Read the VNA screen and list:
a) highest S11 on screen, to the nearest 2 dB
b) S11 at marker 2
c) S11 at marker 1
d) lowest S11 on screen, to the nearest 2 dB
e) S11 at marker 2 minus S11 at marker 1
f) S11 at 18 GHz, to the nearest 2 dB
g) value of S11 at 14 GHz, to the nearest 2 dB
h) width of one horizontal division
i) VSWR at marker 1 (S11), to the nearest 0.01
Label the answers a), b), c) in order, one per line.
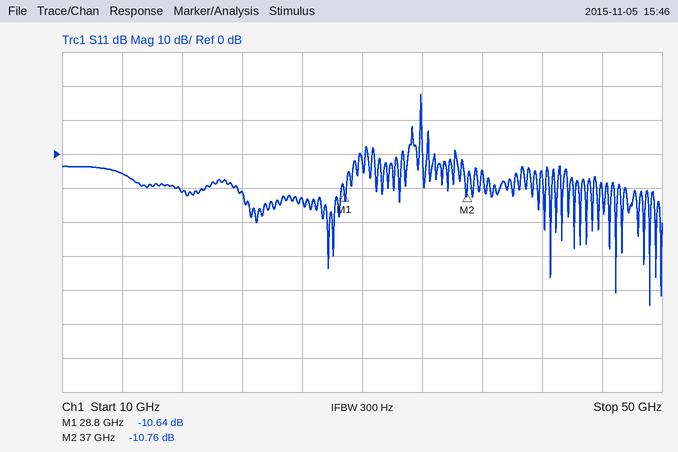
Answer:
a) 18 dB
b) -10.76 dB
c) -10.64 dB
d) -44 dB
e) -0.12 dB
f) -12 dB
g) -6 dB
h) 4 GHz
i) 1.83
